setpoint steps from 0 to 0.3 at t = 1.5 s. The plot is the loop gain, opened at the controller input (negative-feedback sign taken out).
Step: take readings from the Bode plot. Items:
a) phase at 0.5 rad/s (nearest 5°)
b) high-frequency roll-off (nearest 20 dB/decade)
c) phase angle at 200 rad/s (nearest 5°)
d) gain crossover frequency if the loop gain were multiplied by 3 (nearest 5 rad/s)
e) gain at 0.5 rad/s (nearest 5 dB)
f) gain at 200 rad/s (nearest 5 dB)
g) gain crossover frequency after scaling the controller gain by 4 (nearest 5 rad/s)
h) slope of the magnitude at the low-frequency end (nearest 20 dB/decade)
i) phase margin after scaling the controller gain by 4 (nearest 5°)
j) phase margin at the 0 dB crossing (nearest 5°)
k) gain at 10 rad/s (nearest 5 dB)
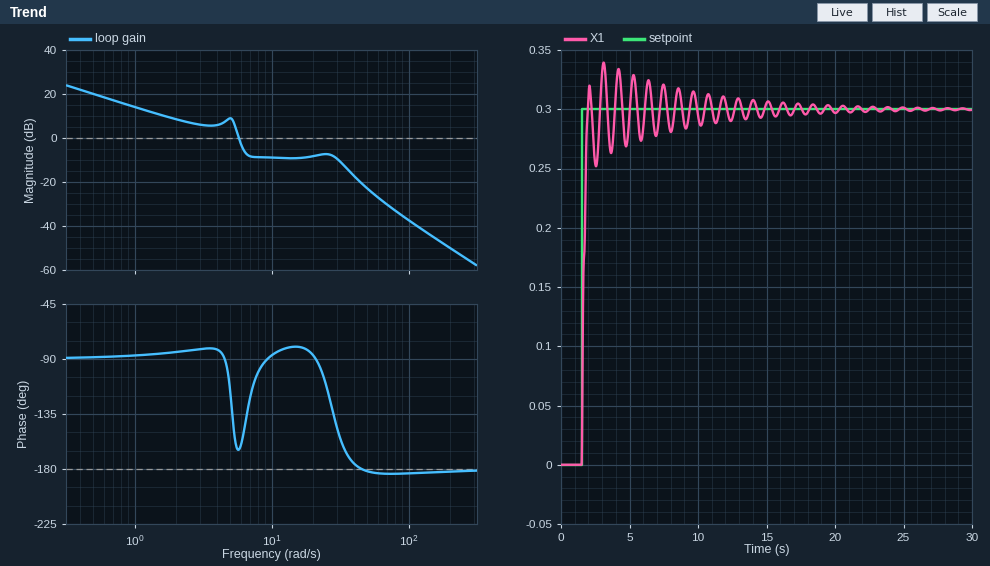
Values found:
-90°
-40 dB/decade
-180°
30 rad/s
20 dB
-50 dB
35 rad/s
-20 dB/decade
20°
15°
-10 dB
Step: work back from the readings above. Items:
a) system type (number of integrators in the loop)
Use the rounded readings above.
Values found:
1
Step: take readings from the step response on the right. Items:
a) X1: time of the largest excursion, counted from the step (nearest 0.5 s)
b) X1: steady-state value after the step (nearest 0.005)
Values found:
1.5 s
0.300
